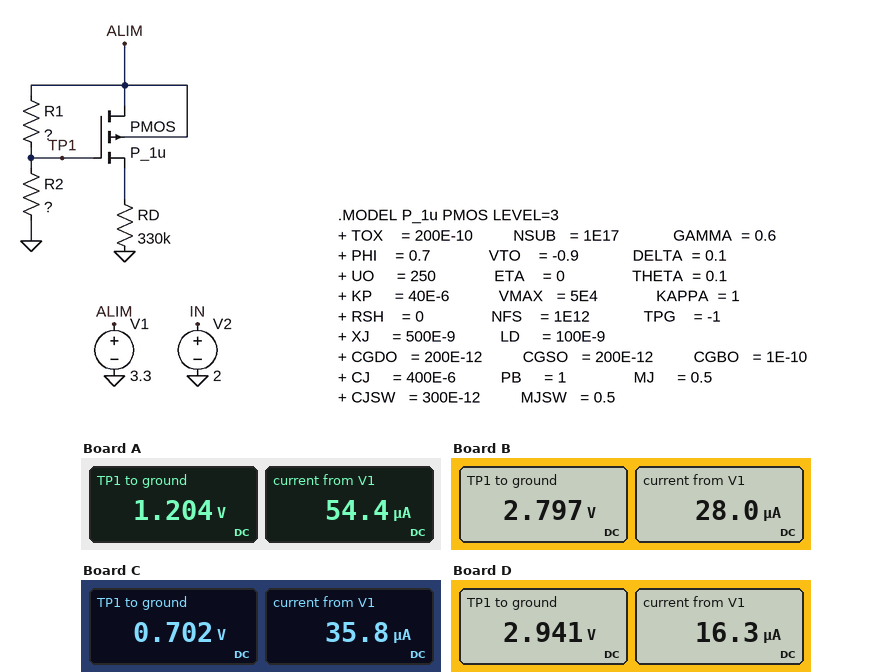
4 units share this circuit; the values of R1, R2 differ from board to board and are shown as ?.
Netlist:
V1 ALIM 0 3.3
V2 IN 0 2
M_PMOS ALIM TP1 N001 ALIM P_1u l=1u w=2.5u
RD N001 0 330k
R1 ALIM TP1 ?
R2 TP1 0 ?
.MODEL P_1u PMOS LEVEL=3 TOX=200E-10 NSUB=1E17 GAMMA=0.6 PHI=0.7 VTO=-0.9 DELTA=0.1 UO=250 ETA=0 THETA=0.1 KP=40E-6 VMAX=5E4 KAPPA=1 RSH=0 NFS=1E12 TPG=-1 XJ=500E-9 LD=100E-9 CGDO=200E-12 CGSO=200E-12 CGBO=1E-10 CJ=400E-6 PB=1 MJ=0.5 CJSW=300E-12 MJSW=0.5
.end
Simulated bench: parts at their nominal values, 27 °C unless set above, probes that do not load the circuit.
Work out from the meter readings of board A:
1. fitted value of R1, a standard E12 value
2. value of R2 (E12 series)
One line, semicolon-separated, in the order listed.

47 kΩ; 27 kΩ
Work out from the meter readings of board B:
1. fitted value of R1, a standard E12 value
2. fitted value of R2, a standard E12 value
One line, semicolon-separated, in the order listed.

18 kΩ; 100 kΩ
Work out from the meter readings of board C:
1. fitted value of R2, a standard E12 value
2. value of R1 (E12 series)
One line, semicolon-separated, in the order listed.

27 kΩ; 100 kΩ
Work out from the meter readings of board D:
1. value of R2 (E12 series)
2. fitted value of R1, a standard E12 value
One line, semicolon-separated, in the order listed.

180 kΩ; 22 kΩ
